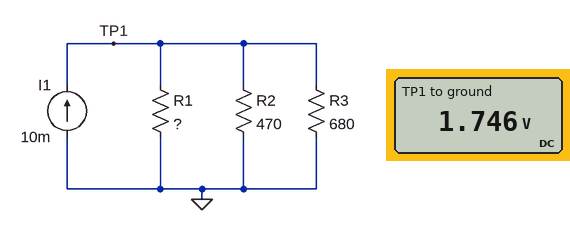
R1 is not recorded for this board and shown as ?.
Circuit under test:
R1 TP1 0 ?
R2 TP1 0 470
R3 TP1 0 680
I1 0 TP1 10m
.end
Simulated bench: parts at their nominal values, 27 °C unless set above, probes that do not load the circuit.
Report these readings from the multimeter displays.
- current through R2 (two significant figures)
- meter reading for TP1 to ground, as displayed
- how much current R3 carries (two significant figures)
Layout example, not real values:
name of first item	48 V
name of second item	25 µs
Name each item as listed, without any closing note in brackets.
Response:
current through R2	3.7 mA
meter reading for TP1 to ground, as displayed	1.746 V
how much current R3 carries	2.6 mA
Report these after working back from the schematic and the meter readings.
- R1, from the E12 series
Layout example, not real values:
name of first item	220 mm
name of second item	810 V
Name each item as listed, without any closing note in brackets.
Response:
R1, from the E12 series	470 Ω
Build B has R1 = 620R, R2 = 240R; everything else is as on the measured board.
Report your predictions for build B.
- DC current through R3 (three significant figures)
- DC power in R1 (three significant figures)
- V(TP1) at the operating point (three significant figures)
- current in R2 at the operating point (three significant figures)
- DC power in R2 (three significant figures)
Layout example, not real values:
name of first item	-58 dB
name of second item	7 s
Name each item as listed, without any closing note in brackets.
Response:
DC current through R3	2.03 mA
DC power in R1	3.07 mW
V(TP1) at the operating point	1.38 V
current in R2 at the operating point	5.75 mA
DC power in R2	7.93 mW
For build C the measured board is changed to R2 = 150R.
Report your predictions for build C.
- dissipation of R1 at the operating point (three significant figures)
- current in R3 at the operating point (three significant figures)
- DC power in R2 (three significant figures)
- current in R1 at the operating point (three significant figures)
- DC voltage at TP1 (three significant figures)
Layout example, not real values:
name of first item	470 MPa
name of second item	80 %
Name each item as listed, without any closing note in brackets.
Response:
dissipation of R1 at the operating point	2.02 mW
current in R3 at the operating point	1.43 mA
DC power in R2	6.33 mW
current in R1 at the operating point	2.07 mA
DC voltage at TP1	974 mV
